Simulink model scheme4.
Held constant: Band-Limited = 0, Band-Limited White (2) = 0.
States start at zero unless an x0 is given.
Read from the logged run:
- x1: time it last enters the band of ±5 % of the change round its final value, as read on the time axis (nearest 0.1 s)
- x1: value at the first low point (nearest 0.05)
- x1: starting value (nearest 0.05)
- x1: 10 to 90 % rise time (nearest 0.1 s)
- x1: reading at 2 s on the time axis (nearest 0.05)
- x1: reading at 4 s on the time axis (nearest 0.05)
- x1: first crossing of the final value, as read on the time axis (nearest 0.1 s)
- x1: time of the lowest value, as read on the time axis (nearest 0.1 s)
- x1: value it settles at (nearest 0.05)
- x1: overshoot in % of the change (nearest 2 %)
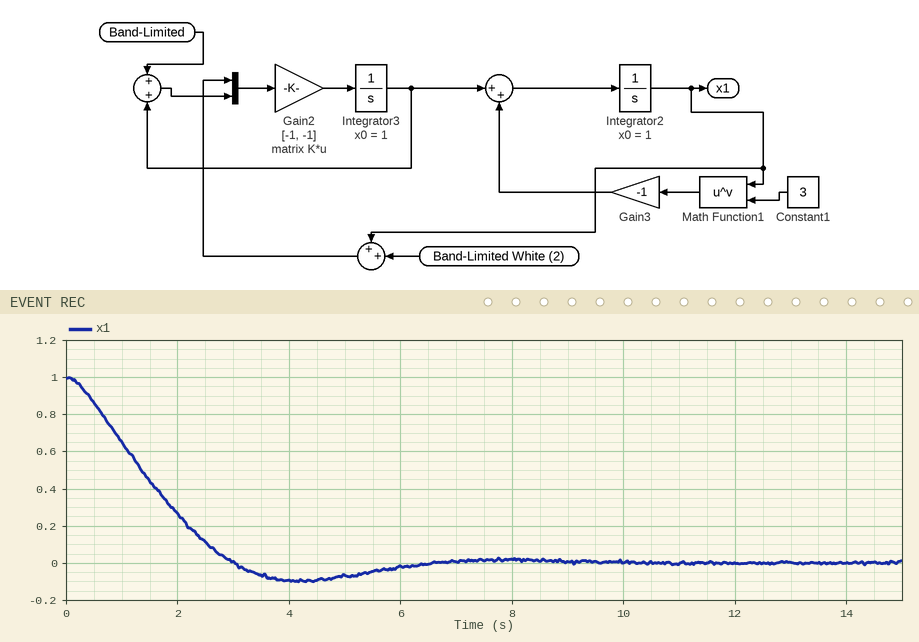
5.5 s
-0.10
1.00
2.1 s
0.25
-0.10
3.0 s
4.2 s
0.00
10 %
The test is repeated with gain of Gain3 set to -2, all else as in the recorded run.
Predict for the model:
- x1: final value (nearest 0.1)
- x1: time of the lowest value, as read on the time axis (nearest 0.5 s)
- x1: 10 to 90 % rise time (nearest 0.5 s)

0.0
4.5 s
2.5 s
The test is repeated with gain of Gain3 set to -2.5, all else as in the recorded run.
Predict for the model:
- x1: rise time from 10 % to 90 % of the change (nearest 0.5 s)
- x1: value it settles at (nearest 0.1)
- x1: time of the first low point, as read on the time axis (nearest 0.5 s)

2.5 s
0.0
4.5 s
